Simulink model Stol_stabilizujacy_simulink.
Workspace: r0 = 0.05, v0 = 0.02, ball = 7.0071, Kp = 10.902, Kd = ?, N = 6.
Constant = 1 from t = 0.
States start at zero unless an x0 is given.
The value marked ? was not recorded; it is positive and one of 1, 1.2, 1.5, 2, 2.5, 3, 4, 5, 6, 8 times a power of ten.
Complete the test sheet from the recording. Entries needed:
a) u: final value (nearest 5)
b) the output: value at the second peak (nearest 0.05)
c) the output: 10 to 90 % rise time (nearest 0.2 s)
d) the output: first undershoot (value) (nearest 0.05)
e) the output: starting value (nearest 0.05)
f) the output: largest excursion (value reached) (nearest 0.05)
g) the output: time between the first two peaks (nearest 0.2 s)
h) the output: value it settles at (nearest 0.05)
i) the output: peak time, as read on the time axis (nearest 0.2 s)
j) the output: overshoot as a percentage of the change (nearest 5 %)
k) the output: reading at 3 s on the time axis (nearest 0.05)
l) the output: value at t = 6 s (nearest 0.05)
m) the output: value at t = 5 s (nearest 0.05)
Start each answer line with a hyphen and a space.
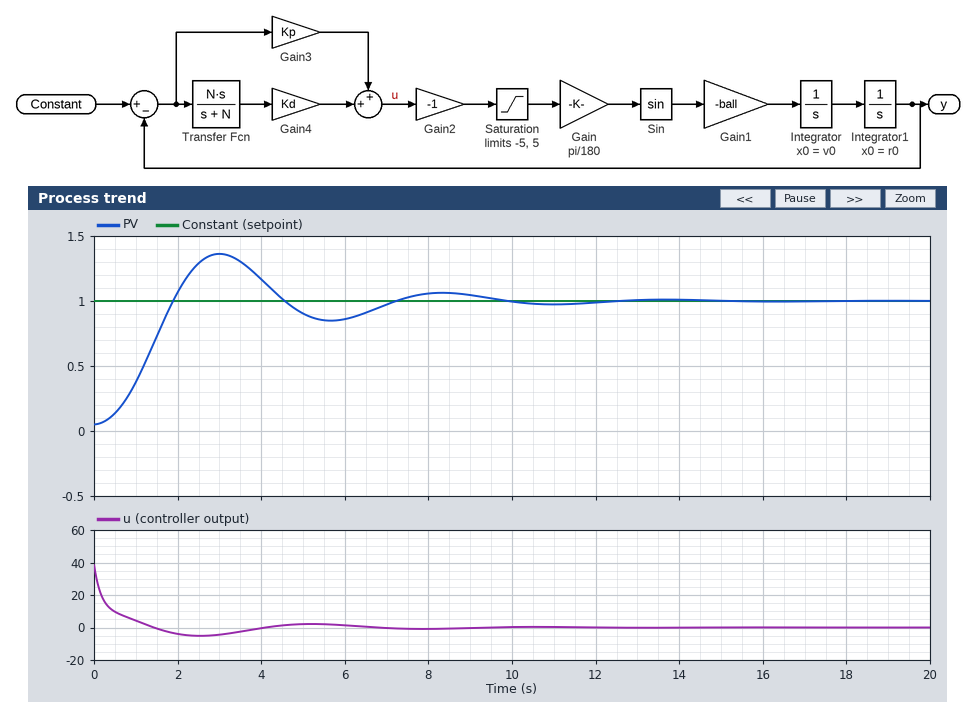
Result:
- 0
- 1.05
- 1.2 s
- 0.85
- 0.05
- 1.35
- 5.4 s
- 1.00
- 3.0 s
- 40 %
- 1.35
- 0.85
- 0.90
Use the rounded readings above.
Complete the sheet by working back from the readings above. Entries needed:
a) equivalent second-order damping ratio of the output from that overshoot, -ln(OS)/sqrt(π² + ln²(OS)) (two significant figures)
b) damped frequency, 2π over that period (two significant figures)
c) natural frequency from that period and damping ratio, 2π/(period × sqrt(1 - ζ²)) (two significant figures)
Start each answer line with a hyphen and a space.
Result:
- 0.28
- 1.2 rad/s
- 1.2 rad/s
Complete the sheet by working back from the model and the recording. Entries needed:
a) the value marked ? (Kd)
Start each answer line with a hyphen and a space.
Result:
- 5
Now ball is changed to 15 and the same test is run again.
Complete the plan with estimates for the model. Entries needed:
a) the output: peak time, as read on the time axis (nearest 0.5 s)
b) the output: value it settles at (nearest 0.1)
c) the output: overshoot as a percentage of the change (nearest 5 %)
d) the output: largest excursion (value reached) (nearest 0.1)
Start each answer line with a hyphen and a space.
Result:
- 2.0 s
- 1.0
- 25 %
- 1.2
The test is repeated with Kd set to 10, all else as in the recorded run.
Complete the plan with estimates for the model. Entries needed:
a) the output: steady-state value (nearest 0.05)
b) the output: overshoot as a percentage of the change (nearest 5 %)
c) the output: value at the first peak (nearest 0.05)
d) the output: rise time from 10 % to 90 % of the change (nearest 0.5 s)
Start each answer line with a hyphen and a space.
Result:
- 1.00
- 10 %
- 1.10
- 1.5 s
